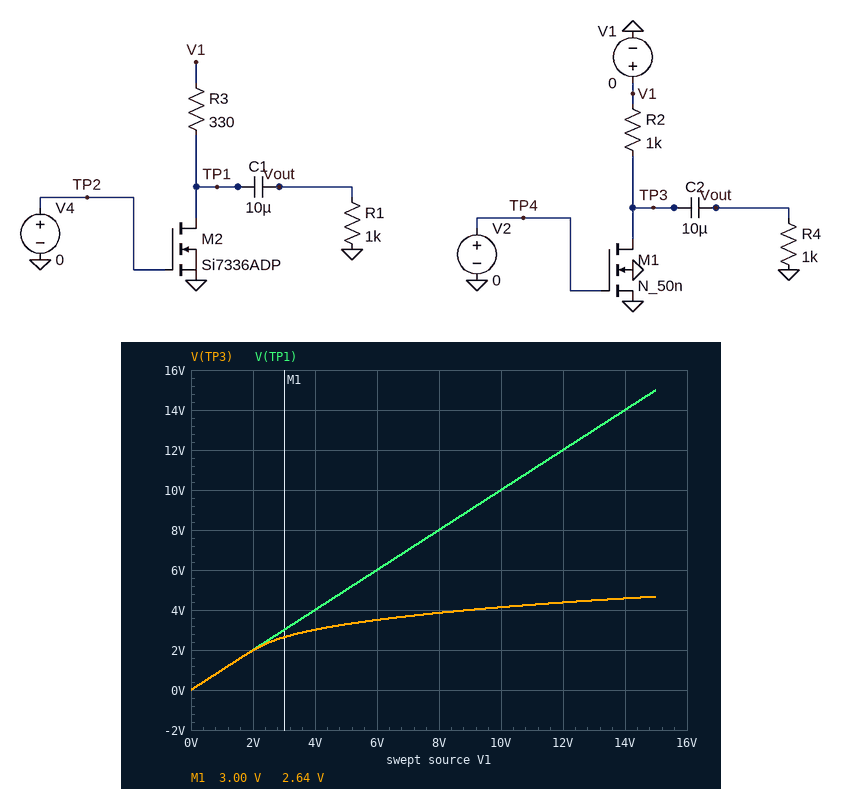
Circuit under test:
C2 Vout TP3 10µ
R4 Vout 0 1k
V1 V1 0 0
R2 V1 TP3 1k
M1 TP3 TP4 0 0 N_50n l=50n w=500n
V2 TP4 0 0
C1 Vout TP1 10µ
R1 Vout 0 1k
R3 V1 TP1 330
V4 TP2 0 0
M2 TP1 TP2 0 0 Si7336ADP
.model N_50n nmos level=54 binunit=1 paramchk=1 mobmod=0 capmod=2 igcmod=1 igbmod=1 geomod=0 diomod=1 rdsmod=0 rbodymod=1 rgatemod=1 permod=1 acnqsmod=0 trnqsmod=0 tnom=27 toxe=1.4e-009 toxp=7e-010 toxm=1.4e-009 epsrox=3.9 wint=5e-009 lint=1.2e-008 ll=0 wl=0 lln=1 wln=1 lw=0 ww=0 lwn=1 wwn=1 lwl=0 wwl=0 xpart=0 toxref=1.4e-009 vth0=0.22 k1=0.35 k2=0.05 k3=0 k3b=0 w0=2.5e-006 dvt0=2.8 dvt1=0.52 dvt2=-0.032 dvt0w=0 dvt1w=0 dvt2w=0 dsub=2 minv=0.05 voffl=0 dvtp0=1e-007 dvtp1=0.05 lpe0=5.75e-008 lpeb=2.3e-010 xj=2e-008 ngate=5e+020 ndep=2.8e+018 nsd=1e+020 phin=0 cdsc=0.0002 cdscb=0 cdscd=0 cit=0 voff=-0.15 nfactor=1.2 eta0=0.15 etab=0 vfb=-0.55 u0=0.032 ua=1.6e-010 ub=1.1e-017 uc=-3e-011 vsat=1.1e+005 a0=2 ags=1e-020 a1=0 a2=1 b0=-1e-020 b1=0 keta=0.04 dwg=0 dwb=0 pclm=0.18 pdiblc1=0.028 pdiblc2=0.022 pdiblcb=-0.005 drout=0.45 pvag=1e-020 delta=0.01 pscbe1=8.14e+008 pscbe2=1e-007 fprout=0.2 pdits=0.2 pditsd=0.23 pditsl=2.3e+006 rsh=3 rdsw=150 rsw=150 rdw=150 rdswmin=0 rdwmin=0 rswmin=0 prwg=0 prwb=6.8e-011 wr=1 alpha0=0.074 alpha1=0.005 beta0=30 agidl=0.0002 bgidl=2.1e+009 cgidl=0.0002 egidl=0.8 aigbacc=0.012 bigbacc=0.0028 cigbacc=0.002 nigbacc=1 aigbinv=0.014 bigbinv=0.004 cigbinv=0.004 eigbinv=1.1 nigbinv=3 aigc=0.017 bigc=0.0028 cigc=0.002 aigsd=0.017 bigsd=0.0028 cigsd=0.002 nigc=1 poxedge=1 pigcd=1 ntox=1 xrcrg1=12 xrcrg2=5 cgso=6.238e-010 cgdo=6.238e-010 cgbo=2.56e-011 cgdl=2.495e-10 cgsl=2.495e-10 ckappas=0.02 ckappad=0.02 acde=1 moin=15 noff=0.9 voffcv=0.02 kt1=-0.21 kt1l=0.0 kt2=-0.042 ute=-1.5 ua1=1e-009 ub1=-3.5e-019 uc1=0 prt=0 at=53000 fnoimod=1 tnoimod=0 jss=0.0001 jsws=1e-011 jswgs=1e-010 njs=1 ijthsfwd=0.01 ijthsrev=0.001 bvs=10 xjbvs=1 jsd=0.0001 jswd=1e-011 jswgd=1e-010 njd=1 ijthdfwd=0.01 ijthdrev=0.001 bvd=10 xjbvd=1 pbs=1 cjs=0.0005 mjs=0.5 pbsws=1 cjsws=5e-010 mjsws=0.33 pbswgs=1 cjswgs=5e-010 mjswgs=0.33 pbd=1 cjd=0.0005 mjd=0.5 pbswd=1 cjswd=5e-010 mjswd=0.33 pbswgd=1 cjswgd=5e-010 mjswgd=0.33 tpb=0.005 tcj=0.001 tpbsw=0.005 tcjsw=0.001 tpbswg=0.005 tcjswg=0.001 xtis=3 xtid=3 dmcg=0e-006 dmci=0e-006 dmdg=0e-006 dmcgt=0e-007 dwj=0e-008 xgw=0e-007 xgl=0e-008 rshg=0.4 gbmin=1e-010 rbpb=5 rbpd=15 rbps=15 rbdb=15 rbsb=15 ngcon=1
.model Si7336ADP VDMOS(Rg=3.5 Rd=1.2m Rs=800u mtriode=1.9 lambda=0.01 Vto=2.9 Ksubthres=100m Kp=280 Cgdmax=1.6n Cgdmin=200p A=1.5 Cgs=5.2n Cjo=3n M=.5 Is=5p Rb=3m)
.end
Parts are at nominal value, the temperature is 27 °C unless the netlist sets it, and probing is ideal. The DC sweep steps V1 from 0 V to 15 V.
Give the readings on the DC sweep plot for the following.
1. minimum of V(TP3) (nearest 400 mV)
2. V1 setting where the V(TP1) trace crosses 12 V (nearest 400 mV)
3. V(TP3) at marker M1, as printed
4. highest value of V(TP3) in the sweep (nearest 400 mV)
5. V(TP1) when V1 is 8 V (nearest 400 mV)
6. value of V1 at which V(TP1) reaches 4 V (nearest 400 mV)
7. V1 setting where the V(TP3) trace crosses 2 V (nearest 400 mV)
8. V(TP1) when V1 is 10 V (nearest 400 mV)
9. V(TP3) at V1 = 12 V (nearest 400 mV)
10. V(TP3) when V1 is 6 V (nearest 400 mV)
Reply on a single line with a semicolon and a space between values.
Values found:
0 V; 12.0 V; 2.64 V; 4.8 V; 8.0 V; 4.0 V; 2.0 V; 10.0 V; 4.4 V; 3.6 V
